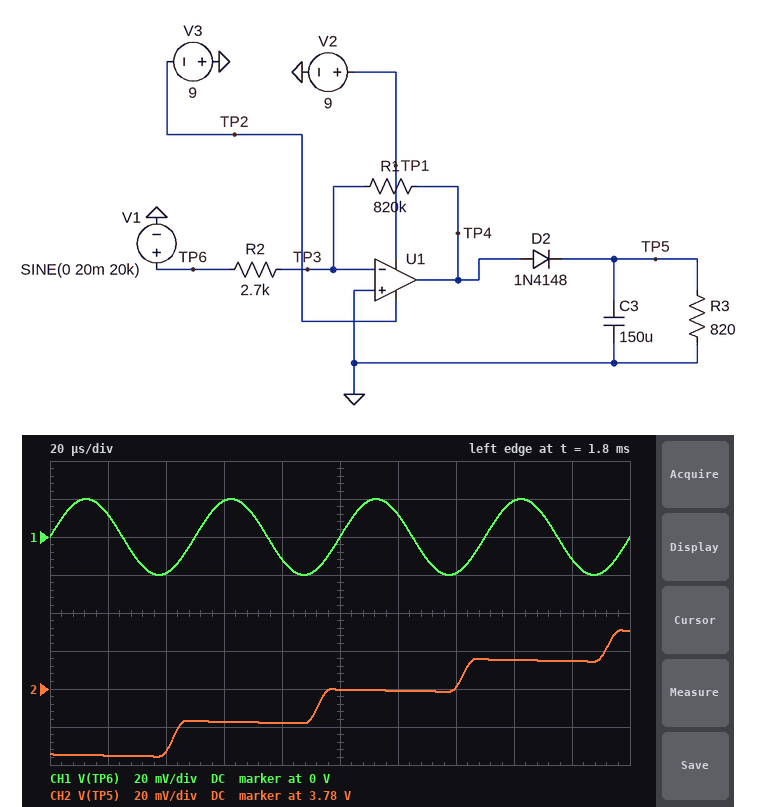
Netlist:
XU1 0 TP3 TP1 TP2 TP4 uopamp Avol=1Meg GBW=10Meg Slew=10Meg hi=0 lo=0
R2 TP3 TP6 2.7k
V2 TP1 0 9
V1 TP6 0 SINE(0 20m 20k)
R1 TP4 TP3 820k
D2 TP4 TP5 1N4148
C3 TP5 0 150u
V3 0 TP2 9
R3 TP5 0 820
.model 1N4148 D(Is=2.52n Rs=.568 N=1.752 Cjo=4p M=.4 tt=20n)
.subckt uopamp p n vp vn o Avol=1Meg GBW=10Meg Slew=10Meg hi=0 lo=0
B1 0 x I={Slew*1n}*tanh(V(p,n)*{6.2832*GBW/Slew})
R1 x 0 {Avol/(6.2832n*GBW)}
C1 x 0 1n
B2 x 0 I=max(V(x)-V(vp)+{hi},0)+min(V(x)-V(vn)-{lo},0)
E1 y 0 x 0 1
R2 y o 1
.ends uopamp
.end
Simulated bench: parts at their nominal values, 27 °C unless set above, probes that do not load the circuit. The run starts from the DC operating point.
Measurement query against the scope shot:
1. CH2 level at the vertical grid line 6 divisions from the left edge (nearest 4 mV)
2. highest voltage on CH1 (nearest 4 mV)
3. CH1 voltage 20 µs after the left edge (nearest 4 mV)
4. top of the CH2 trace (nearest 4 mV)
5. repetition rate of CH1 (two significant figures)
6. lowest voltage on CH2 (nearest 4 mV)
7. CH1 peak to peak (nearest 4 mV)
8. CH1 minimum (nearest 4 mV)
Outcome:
3.780 V
20 mV
12 mV
3.812 V
20 kHz
3.744 V
40 mV
-20 mV
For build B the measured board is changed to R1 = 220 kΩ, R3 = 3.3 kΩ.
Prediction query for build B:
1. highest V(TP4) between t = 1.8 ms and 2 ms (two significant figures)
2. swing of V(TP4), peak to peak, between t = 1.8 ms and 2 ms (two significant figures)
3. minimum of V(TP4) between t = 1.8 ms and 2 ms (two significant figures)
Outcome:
1.6 V
3.2 V
-1.6 V
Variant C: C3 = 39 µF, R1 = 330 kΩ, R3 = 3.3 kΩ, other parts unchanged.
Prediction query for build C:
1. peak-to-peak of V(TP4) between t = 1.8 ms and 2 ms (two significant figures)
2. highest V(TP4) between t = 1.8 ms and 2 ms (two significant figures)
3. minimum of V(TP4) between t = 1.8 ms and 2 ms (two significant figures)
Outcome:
4.7 V
2.4 V
-2.4 V
